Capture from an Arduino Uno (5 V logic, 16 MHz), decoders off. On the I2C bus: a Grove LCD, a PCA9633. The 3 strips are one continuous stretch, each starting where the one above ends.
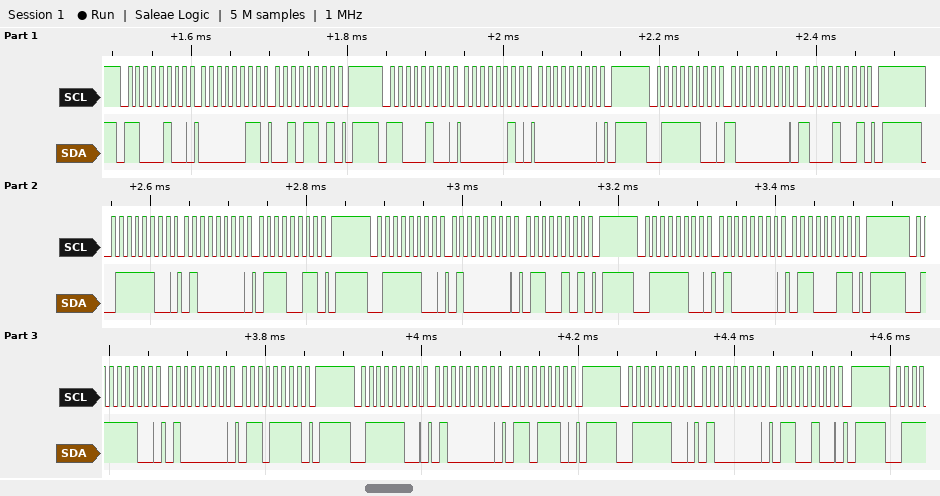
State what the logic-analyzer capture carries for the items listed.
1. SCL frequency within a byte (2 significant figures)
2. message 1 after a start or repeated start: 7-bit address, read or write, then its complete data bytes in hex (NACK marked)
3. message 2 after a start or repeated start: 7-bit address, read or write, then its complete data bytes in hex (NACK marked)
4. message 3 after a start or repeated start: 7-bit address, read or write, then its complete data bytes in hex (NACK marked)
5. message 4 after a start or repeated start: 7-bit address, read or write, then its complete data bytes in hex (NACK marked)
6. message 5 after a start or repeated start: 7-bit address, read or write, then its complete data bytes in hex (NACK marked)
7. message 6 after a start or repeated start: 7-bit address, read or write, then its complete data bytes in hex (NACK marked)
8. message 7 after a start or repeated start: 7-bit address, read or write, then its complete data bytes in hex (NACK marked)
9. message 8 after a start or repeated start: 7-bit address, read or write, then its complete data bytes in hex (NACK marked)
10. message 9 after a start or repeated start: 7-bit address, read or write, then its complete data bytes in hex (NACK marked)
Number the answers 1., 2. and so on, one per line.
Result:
1. 100 kHz
2. 0x62 write: 03 2D
3. 0x62 write: 02 00
4. 0x3E write: 80 89
5. 0x3E write: 40 73
6. 0x3E write: 40 65
7. 0x3E write: 40 63
8. 0x3E write: 40 6F
9. 0x3E write: 40 6E
10. 0x3E write: 40 64
